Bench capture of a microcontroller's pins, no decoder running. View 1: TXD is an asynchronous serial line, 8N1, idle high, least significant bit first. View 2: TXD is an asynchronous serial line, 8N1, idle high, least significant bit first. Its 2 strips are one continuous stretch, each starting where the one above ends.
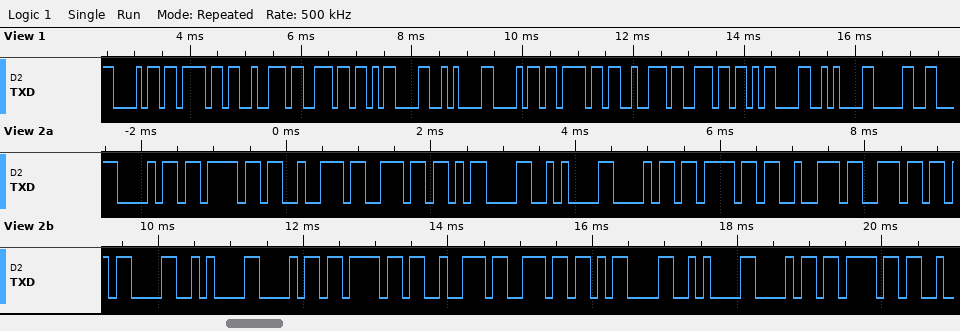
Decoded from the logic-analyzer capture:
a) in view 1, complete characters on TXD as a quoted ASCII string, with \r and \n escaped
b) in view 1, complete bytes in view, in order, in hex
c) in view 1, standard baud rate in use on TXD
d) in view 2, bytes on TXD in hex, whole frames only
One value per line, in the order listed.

"horn\r\nhorn\r\n0"
68 6F 72 6E 0D 0A 68 6F 72 6E 0D 0A 30
9600 baud
68 6F 72 6E 0D 0A 68 6F 72 6E 0D 0A 68 6F 72 6E 0D 0A 68 6F
